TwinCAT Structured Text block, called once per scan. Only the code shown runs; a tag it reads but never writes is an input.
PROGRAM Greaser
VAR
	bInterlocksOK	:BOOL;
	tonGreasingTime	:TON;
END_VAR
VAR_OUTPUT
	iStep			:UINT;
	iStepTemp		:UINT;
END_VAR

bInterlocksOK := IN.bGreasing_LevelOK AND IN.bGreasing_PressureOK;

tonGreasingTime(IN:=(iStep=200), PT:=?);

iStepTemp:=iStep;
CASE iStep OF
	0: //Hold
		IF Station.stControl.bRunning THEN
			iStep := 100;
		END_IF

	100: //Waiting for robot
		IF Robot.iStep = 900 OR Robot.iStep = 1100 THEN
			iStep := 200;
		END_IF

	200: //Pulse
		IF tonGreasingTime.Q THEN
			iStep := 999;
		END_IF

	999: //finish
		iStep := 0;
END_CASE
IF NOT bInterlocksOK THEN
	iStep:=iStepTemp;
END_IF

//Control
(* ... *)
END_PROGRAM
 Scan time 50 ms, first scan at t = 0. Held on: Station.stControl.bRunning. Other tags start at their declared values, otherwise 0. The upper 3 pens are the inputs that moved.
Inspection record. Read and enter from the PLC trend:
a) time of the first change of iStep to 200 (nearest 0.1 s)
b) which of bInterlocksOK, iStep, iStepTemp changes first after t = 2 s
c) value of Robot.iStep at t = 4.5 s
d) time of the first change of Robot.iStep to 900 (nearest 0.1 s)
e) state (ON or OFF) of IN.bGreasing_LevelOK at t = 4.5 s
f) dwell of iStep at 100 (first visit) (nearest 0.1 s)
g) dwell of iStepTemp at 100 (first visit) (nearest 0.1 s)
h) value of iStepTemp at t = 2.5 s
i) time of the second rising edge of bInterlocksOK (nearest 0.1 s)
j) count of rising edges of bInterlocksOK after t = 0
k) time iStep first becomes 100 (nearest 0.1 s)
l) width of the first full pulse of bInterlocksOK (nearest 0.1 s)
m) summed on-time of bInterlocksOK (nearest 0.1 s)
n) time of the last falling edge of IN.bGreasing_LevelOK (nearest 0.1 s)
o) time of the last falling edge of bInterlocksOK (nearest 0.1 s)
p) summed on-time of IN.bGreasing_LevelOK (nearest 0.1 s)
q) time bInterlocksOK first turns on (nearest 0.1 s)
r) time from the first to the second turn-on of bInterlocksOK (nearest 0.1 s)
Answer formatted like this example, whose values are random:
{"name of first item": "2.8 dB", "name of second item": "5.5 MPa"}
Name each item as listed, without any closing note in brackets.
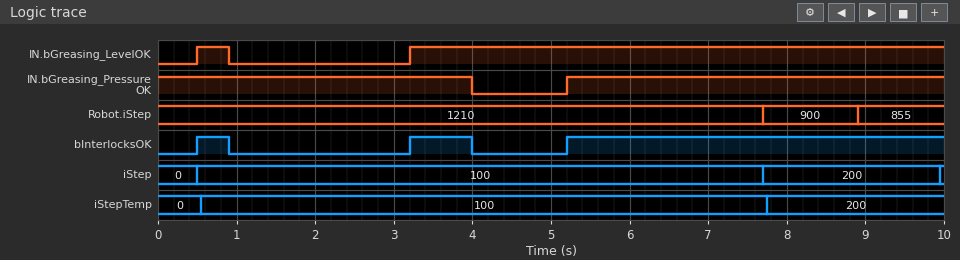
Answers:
{"time of the first change of iStep to 200": "7.7 s", "which of bInterlocksOK, iStep, iStepTemp changes first after t = 2 s": "bInterlocksOK", "value of Robot.iStep at t = 4.5 s": "1210", "time of the first change of Robot.iStep to 900": "7.7 s", "state (ON or OFF) of IN.bGreasing_LevelOK at t = 4.5 s": "ON", "dwell of iStep at 100 (first visit)": "7.2 s", "dwell of iStepTemp at 100 (first visit)": "7.2 s", "value of iStepTemp at t = 2.5 s": "100", "time of the second rising edge of bInterlocksOK": "3.2 s", "count of rising edges of bInterlocksOK after t = 0": "3", "time iStep first becomes 100": "0.5 s", "width of the first full pulse of bInterlocksOK": "0.4 s", "summed on-time of bInterlocksOK": "6.0 s", "time of the last falling edge of IN.bGreasing_LevelOK": "0.9 s", "time of the last falling edge of bInterlocksOK": "4.0 s", "summed on-time of IN.bGreasing_LevelOK": "7.2 s", "time bInterlocksOK first turns on": "0.5 s", "time from the first to the second turn-on of bInterlocksOK": "2.7 s"}
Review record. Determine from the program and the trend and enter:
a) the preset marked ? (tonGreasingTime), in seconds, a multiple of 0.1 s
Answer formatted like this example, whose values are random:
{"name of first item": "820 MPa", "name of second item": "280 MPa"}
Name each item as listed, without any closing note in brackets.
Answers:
{"the preset marked ? (tonGreasingTime), in seconds, a multiple of 0.1 s": "2.2 s"}
